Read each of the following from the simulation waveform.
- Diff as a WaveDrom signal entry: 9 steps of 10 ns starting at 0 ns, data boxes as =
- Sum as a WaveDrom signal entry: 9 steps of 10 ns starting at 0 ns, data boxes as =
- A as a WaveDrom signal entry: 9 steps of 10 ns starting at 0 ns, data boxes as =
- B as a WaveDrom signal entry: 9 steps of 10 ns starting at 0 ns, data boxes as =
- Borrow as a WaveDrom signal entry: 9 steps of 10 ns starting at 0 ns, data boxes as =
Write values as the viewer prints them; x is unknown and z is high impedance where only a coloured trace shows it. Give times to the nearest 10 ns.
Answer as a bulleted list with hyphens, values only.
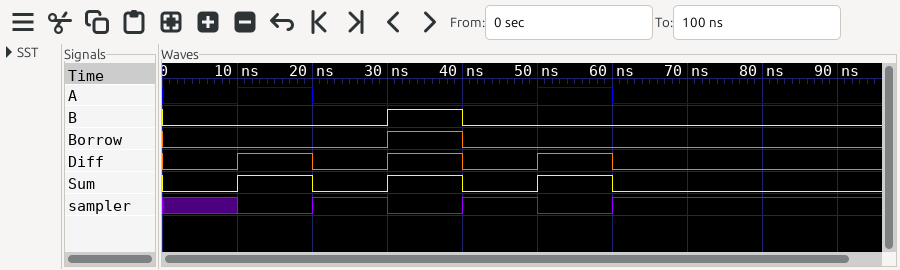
- {name: 'Diff', wave: '0101010..'}
- {name: 'Sum', wave: '0101010..'}
- {name: 'A', wave: '010..10..'}
- {name: 'B', wave: '0..10....'}
- {name: 'Borrow', wave: '0..10....'}
